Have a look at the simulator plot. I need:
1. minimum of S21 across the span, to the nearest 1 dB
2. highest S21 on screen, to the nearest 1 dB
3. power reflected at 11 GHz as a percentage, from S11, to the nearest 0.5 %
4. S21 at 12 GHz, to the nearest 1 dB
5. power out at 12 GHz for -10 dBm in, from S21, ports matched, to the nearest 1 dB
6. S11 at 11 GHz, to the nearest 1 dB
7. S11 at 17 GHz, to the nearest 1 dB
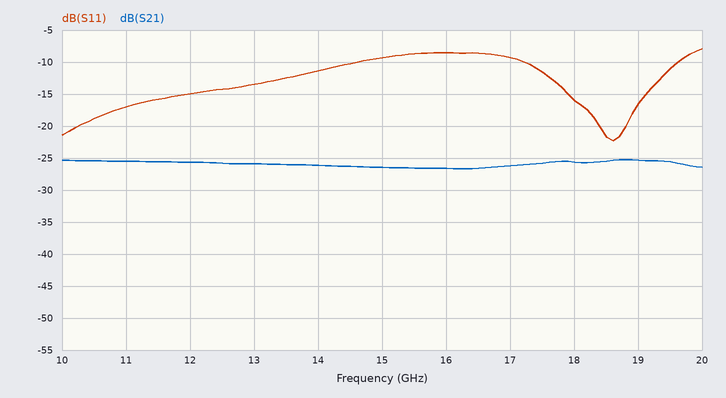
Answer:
-27 dB
-25 dB
2.0 %
-26 dB
-36 dBm
-17 dB
-9 dB
